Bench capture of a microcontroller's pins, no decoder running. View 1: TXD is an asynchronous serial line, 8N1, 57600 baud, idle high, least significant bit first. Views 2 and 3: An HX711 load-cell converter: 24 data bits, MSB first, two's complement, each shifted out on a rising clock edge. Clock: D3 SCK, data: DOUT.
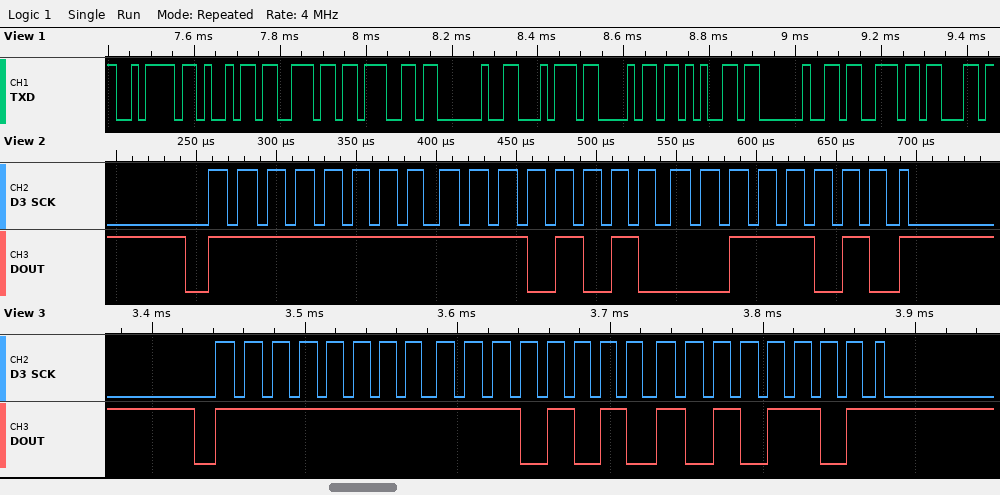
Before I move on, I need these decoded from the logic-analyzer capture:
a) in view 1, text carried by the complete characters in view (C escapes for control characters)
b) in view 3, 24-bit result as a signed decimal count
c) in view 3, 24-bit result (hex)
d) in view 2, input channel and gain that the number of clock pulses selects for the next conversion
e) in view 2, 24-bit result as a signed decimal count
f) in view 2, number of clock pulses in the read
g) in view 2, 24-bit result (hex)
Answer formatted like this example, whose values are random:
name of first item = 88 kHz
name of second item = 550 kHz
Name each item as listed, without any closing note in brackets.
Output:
in view 1, text carried by the complete characters in view = "zing the sc"
in view 3, 24-bit result as a signed decimal count = -5459
in view 3, 24-bit result = 0xFFEAAD
in view 2, input channel and gain that the number of clock pulses selects for the next conversion = channel A, gain 128
in view 2, 24-bit result as a signed decimal count = -5574
in view 2, number of clock pulses in the read = 25
in view 2, 24-bit result = 0xFFEA3A
